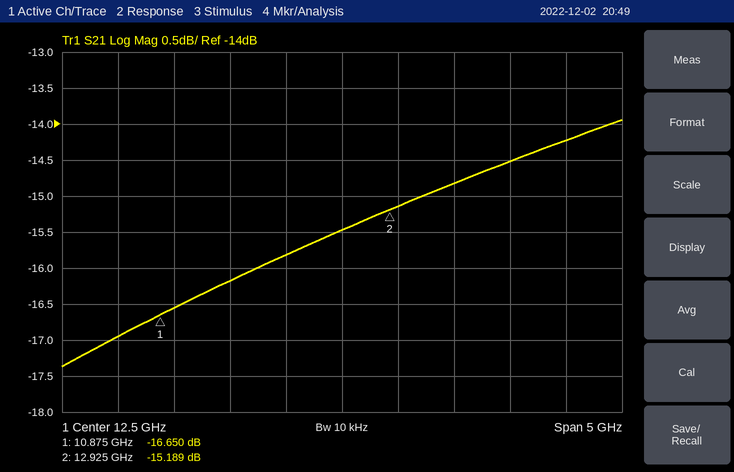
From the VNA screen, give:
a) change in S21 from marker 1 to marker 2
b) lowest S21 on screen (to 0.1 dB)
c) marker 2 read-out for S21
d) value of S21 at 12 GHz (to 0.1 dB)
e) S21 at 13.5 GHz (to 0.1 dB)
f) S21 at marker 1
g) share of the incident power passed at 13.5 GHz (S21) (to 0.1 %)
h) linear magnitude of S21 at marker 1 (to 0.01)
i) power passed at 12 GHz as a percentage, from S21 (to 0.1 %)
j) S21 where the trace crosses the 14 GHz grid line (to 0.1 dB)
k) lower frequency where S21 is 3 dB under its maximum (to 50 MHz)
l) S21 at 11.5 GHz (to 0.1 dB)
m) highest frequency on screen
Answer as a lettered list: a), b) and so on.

a) 1.461 dB
b) -17.4 dB
c) -15.189 dB
d) -15.8 dB
e) -14.8 dB
f) -16.650 dB
g) 3.3 %
h) 0.15
i) 2.6 %
j) -14.5 dB
k) 10.50 GHz
l) -16.2 dB
m) 15 GHz
